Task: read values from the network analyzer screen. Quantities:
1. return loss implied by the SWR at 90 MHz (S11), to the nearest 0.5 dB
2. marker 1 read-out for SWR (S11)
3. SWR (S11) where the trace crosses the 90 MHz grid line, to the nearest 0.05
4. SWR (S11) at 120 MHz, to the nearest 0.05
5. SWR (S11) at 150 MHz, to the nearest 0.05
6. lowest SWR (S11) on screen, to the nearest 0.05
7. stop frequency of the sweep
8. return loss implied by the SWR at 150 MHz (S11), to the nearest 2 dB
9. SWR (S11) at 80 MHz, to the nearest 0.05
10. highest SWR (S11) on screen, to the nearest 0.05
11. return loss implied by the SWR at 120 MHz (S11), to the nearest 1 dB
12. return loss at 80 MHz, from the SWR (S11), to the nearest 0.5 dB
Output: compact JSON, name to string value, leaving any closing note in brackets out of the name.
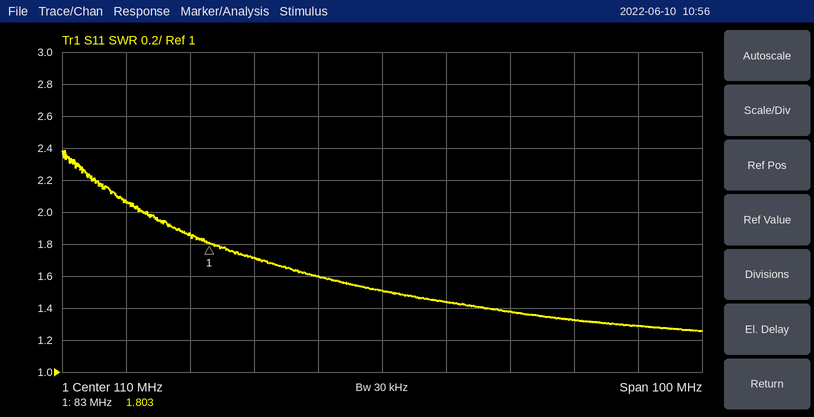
{"return loss implied by the SWR at 90 MHz (S11), to the nearest 0.5 dB": "11.5 dB", "marker 1 read-out for SWR": "1.803", "SWR (S11) where the trace crosses the 90 MHz grid line, to the nearest 0.05": "1.70", "SWR (S11) at 120 MHz, to the nearest 0.05": "1.45", "SWR (S11) at 150 MHz, to the nearest 0.05": "1.30", "lowest SWR (S11) on screen, to the nearest 0.05": "1.25", "stop frequency of the sweep": "160 MHz", "return loss implied by the SWR at 150 MHz (S11), to the nearest 2 dB": "18 dB", "SWR (S11) at 80 MHz, to the nearest 0.05": "1.85", "highest SWR (S11) on screen, to the nearest 0.05": "2.40", "return loss implied by the SWR at 120 MHz (S11), to the nearest 1 dB": "15 dB", "return loss at 80 MHz, from the SWR (S11), to the nearest 0.5 dB": "10.5 dB"}
